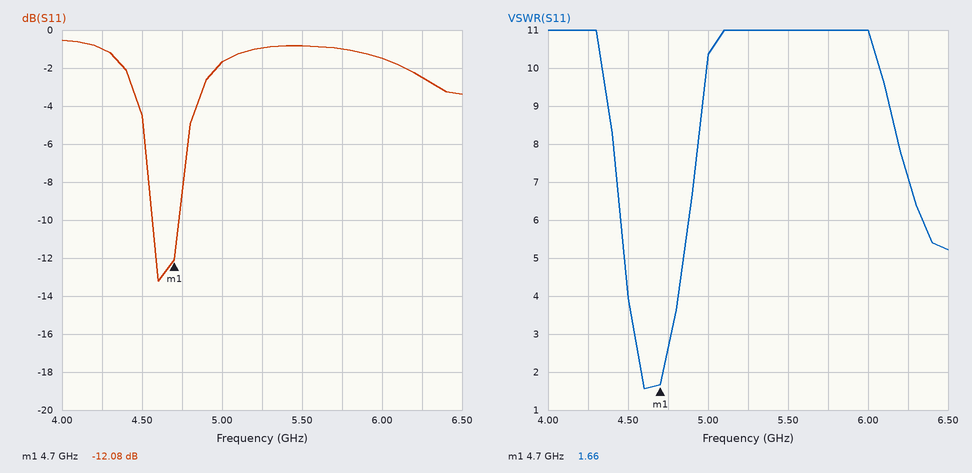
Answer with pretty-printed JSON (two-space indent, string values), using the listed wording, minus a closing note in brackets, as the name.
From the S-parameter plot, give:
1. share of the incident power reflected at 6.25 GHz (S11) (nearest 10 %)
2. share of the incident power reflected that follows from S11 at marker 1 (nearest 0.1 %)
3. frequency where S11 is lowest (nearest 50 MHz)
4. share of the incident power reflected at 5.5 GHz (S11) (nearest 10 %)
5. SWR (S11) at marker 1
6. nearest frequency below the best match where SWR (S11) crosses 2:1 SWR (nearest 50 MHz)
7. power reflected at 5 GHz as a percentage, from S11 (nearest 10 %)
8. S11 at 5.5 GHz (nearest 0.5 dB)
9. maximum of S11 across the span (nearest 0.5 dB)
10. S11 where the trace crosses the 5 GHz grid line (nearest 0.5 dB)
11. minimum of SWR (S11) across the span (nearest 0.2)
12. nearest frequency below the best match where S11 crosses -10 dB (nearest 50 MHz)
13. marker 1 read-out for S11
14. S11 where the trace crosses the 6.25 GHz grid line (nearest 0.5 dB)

{
  "share of the incident power reflected at 6.25 GHz (S11)": "60 %",
  "share of the incident power reflected that follows from S11 at marker 1": "6.2 %",
  "frequency where S11 is lowest": "4.60 GHz",
  "share of the incident power reflected at 5.5 GHz (S11)": "80 %",
  "SWR (S11) at marker 1": "1.66",
  "nearest frequency below the best match where SWR (S11) crosses 2:1 SWR": "4.60 GHz",
  "power reflected at 5 GHz as a percentage, from S11": "70 %",
  "S11 at 5.5 GHz": "-1.0 dB",
  "maximum of S11 across the span": "-0.5 dB",
  "S11 where the trace crosses the 5 GHz grid line": "-1.5 dB",
  "minimum of SWR (S11) across the span": "1.6",
  "nearest frequency below the best match where S11 crosses -10 dB": "4.55 GHz",
  "marker 1 read-out for S11": "-12.08 dB",
  "S11 where the trace crosses the 6.25 GHz grid line": "-2.5 dB"
}
